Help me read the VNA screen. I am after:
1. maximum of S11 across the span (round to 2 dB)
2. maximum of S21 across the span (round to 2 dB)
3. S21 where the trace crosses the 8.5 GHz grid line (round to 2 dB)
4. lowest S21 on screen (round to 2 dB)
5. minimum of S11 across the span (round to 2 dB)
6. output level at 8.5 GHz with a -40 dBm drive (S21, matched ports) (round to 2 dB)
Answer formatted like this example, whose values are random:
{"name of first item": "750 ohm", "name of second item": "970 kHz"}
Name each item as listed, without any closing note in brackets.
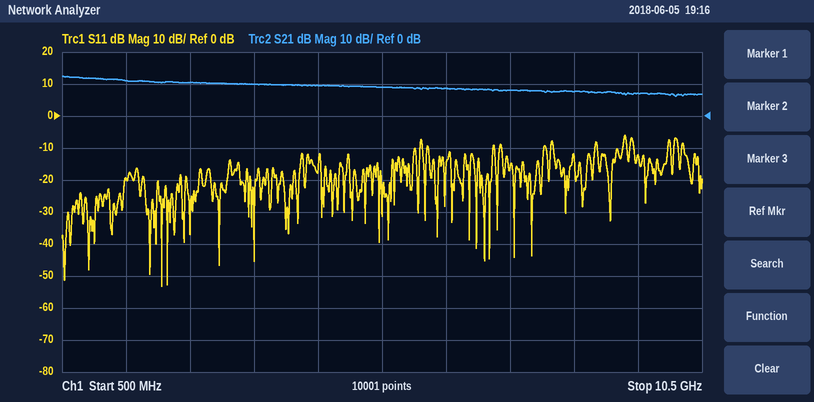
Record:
{"maximum of S11 across the span": "-6 dB", "maximum of S21 across the span": "12 dB", "S21 where the trace crosses the 8.5 GHz grid line": "8 dB", "lowest S21 on screen": "6 dB", "minimum of S11 across the span": "-54 dB", "output level at 8.5 GHz with a -40 dBm drive (S21, matched ports)": "-32 dBm"}
